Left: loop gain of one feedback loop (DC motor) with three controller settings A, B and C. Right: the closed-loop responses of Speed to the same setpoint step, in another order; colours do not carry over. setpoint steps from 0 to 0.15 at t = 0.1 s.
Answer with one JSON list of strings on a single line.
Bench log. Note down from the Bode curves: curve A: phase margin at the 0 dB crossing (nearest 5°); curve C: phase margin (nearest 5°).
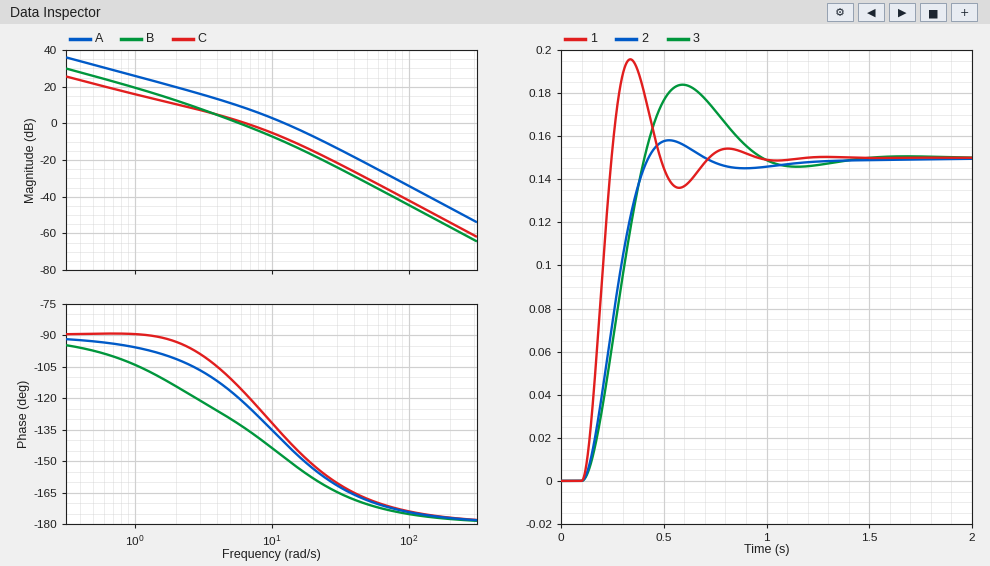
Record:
["40°", "60°"]
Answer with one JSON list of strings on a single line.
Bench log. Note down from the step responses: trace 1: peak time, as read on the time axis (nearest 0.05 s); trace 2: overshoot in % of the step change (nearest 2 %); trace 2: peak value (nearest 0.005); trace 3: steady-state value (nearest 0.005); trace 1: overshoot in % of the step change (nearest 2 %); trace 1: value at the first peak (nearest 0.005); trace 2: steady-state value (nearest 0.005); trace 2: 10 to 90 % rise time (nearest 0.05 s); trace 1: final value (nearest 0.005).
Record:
["0.35 s", "6 %", "0.160", "0.150", "30 %", "0.195", "0.150", "0.20 s", "0.150"]
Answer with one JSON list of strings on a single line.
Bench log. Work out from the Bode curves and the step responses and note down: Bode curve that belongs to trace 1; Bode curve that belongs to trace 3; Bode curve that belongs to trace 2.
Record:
["A", "B", "C"]
